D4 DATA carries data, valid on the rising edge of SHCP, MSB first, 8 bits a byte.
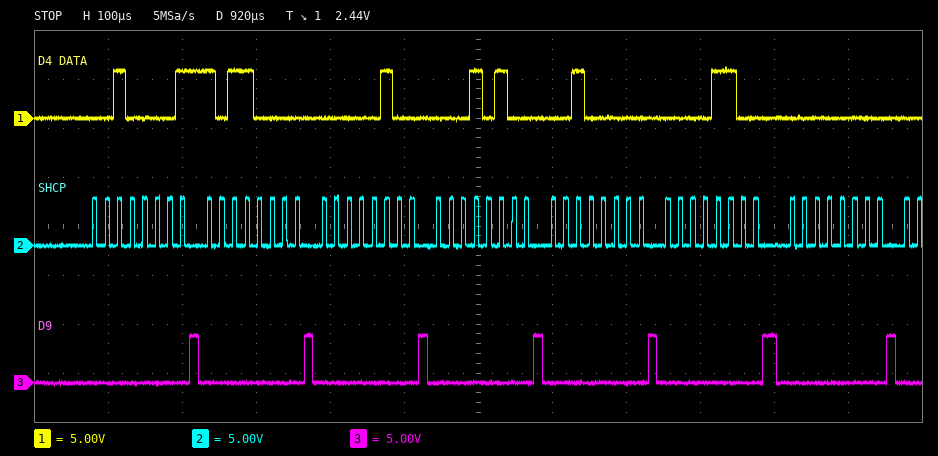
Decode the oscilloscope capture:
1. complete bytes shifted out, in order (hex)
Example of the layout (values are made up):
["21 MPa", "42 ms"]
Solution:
["21 B0 04 14 20 0C 00"]
